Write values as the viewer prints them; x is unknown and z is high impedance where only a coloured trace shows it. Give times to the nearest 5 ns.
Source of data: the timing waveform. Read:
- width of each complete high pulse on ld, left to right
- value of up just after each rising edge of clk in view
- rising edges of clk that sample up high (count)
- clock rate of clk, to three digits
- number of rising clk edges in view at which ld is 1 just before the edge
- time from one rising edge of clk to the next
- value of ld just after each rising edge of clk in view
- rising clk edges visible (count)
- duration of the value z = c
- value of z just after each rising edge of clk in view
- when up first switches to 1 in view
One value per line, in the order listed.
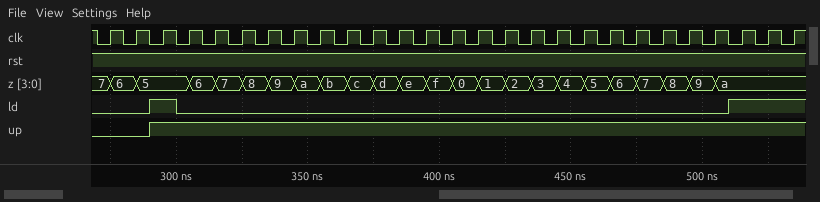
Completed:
10 ns
0 0 1 1 1 1 1 1 1 1 1 1 1 1 1 1 1 1 1 1 1 1 1 1 1 1 1
25
100 MHz
4
10 ns
0 0 1 0 0 0 0 0 0 0 0 0 0 0 0 0 0 0 0 0 0 0 0 0 1 1 1
27
10 ns
6, 5, 5, 6, 7, 8, 9, a, b, c, d, e, f, 0, 1, 2, 3, 4, 5, 6, 7, 8, 9, a, a, a, a
290 ns
